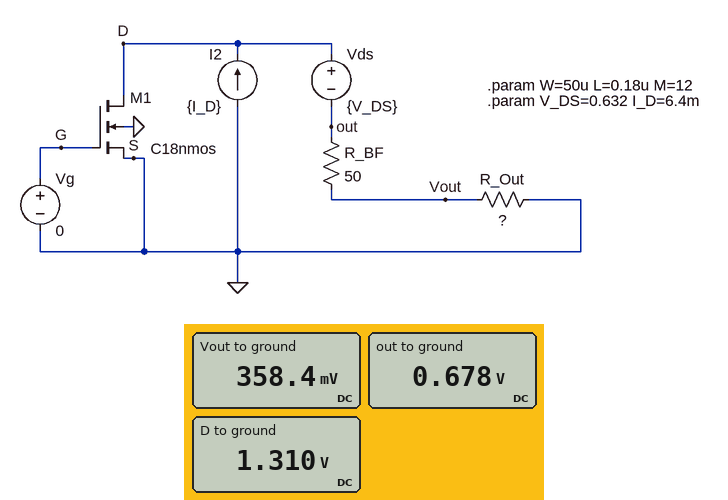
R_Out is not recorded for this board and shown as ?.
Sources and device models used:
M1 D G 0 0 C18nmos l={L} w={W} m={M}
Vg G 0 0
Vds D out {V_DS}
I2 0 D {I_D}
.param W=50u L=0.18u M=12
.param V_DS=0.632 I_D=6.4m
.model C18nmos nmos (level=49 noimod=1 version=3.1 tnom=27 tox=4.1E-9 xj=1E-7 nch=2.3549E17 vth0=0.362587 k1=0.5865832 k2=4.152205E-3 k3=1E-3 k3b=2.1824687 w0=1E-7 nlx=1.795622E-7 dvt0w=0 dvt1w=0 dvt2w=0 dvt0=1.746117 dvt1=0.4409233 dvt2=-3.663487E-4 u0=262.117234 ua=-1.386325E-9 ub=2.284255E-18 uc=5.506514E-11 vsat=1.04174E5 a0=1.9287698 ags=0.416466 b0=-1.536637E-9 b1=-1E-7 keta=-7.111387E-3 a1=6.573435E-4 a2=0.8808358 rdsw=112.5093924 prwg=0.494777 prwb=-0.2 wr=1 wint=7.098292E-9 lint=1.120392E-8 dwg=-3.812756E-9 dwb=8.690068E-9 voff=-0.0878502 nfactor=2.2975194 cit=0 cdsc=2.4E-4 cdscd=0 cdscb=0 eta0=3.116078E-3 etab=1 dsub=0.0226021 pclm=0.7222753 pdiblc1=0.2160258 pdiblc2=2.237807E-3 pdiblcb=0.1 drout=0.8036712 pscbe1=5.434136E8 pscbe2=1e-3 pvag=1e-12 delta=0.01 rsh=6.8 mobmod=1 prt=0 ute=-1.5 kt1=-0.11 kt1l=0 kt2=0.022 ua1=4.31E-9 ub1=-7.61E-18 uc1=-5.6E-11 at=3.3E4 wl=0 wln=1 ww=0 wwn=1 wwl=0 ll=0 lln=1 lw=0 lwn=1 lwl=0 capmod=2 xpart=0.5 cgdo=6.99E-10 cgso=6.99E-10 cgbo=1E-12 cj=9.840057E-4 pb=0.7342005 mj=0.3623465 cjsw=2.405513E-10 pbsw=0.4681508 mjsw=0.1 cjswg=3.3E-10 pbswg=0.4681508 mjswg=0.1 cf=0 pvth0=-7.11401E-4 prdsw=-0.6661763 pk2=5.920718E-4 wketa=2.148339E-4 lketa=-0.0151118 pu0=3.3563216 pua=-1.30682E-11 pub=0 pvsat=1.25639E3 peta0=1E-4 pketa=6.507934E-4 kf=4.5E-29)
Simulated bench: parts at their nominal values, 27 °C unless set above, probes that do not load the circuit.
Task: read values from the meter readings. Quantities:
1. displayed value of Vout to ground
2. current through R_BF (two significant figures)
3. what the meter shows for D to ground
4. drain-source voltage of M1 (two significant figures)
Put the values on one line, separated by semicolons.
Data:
358.4 mV; 6.4 mA; 1.310 V; 1.3 V
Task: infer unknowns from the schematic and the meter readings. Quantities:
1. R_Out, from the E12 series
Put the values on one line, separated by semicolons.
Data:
56 Ω
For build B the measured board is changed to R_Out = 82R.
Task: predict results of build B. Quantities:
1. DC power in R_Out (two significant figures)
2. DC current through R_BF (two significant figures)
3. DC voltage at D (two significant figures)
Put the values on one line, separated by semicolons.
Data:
3.4 mW; 6.4 mA; 1.5 V
